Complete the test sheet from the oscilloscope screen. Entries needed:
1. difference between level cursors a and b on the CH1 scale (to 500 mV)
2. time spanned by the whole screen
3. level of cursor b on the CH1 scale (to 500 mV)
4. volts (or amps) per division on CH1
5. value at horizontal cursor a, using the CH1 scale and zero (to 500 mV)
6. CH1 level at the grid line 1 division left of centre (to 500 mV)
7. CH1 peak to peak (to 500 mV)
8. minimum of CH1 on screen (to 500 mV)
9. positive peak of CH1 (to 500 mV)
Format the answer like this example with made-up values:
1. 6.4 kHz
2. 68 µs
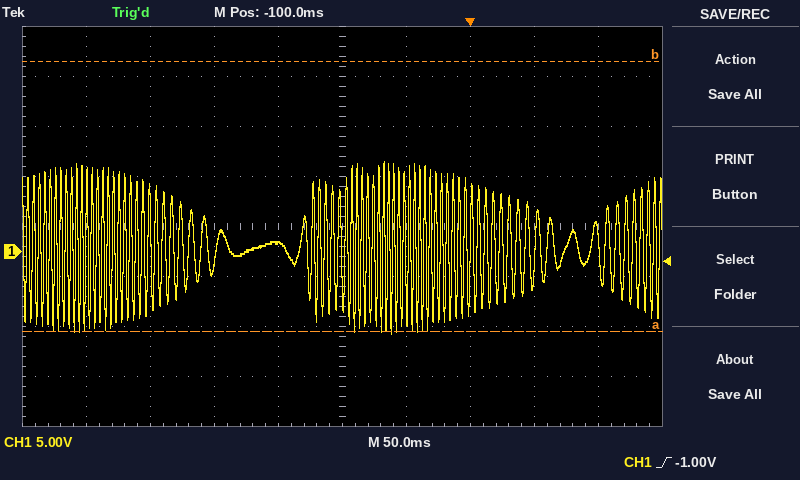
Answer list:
1. 27.0 V
2. 500 ms
3. 19.0 V
4. 5 V
5. -8.0 V
6. 1.0 V
7. 17.0 V
8. -8.0 V
9. 9.0 V
